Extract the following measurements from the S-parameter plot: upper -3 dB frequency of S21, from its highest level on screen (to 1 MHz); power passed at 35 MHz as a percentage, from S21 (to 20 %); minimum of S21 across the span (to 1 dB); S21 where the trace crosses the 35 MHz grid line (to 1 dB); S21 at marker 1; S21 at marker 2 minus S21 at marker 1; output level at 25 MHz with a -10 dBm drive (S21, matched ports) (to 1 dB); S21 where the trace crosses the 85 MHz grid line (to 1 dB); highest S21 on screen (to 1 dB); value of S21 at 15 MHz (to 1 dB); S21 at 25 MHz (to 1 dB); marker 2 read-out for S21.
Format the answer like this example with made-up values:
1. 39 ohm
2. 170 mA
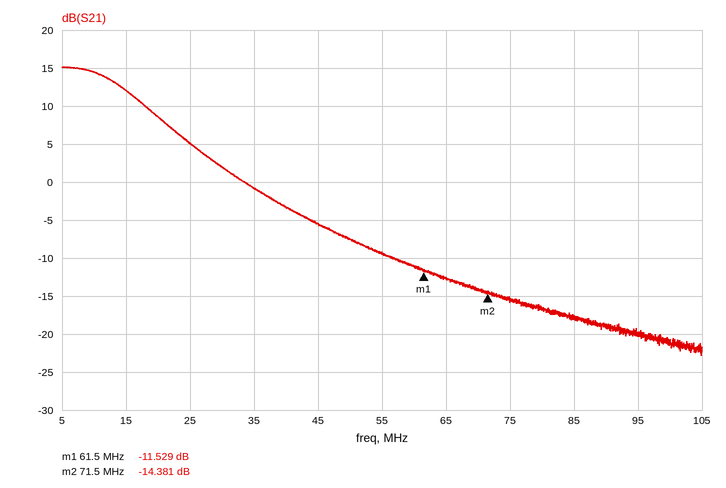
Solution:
1. 15 MHz
2. 80 %
3. -23 dB
4. -1 dB
5. -11.529 dB
6. -2.852 dB
7. -5 dBm
8. -18 dB
9. 15 dB
10. 12 dB
11. 5 dB
12. -14.381 dB
